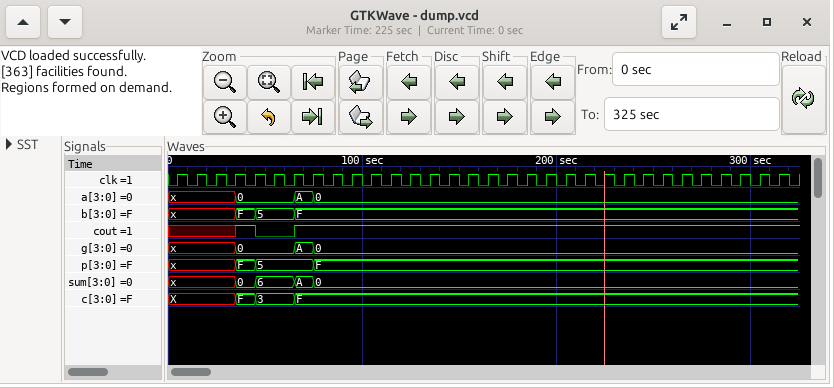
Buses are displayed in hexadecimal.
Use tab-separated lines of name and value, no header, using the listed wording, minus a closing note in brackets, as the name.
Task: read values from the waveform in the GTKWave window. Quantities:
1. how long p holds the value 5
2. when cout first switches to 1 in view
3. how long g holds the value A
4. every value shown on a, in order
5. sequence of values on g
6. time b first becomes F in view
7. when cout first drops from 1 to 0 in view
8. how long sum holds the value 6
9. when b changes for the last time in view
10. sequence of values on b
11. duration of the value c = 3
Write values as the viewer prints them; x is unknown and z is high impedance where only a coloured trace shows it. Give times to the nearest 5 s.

how long p holds the value 5	30 s
when cout first switches to 1 in view	35 s
how long g holds the value A	10 s
every value shown on a, in order	x, 0, A, 0
sequence of values on g	x, 0, A, 0
time b first becomes F in view	35 s
when cout first drops from 1 to 0 in view	45 s
how long sum holds the value 6	20 s
when b changes for the last time in view	65 s
sequence of values on b	x, F, 5, F
duration of the value c = 3	20 s
